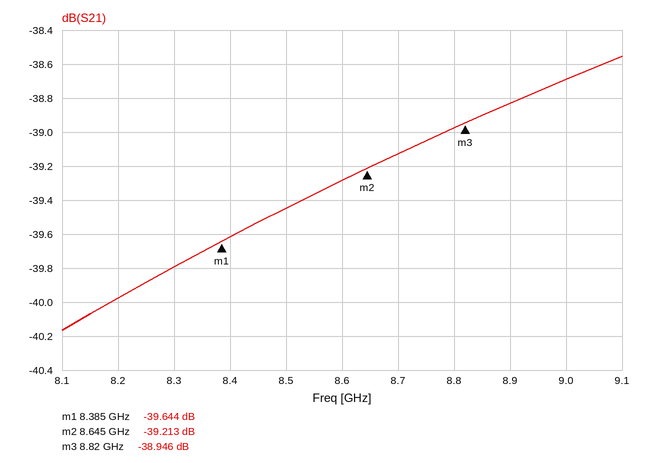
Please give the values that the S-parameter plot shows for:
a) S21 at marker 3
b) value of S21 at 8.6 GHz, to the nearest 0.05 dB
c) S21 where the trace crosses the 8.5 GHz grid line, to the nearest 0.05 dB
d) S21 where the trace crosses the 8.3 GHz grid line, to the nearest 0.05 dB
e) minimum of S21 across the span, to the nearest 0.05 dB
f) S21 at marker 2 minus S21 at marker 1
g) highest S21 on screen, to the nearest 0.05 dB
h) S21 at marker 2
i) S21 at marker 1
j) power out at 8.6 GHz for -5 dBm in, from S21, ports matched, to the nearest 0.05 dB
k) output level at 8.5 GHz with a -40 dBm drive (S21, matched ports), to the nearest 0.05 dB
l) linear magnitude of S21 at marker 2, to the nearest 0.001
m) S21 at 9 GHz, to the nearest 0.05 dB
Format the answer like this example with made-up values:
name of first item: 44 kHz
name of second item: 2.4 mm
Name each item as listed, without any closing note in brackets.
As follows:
S21 at marker 3: -38.946 dB
value of S21 at 8.6 GHz, to the nearest 0.05 dB: -39.30 dB
S21 where the trace crosses the 8.5 GHz grid line, to the nearest 0.05 dB: -39.45 dB
S21 where the trace crosses the 8.3 GHz grid line, to the nearest 0.05 dB: -39.80 dB
minimum of S21 across the span, to the nearest 0.05 dB: -40.15 dB
S21 at marker 2 minus S21 at marker 1: 0.431 dB
highest S21 on screen, to the nearest 0.05 dB: -38.55 dB
S21 at marker 2: -39.213 dB
S21 at marker 1: -39.644 dB
power out at 8.6 GHz for -5 dBm in, from S21, ports matched, to the nearest 0.05 dB: -44.30 dBm
output level at 8.5 GHz with a -40 dBm drive (S21, matched ports), to the nearest 0.05 dB: -79.45 dBm
linear magnitude of S21 at marker 2, to the nearest 0.001: 0.011
S21 at 9 GHz, to the nearest 0.05 dB: -38.70 dB
